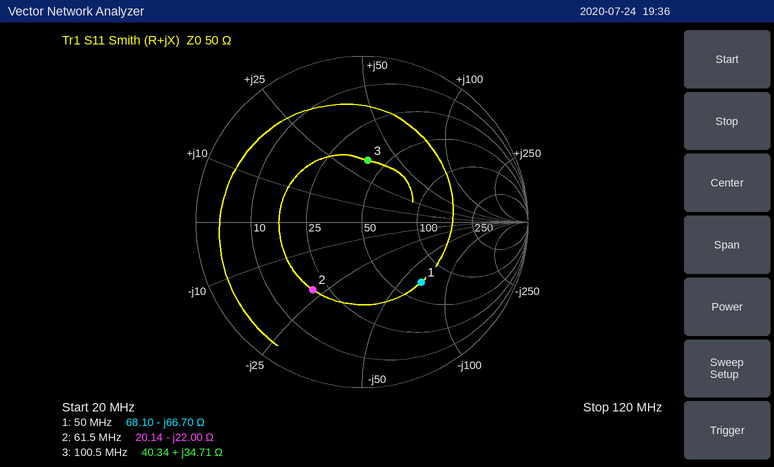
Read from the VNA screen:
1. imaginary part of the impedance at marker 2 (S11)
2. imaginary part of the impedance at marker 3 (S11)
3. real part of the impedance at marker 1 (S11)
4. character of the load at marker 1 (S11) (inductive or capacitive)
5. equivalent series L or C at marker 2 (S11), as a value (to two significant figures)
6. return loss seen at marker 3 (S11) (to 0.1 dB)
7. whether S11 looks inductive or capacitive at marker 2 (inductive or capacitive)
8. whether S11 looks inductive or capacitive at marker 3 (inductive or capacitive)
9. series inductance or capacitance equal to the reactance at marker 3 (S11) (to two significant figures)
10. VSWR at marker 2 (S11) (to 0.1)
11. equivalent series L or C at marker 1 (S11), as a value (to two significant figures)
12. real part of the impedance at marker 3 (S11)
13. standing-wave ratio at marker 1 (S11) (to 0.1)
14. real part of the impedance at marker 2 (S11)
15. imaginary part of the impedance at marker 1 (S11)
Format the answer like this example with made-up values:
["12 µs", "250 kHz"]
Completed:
["-22.00 Ω", "+34.71 Ω", "68.10 Ω", "capacitive", "120 pF", "8.6 dB", "capacitive", "inductive", "55 nH", "3.0", "48 pF", "40.34 Ω", "3.1", "20.14 Ω", "-66.70 Ω"]
